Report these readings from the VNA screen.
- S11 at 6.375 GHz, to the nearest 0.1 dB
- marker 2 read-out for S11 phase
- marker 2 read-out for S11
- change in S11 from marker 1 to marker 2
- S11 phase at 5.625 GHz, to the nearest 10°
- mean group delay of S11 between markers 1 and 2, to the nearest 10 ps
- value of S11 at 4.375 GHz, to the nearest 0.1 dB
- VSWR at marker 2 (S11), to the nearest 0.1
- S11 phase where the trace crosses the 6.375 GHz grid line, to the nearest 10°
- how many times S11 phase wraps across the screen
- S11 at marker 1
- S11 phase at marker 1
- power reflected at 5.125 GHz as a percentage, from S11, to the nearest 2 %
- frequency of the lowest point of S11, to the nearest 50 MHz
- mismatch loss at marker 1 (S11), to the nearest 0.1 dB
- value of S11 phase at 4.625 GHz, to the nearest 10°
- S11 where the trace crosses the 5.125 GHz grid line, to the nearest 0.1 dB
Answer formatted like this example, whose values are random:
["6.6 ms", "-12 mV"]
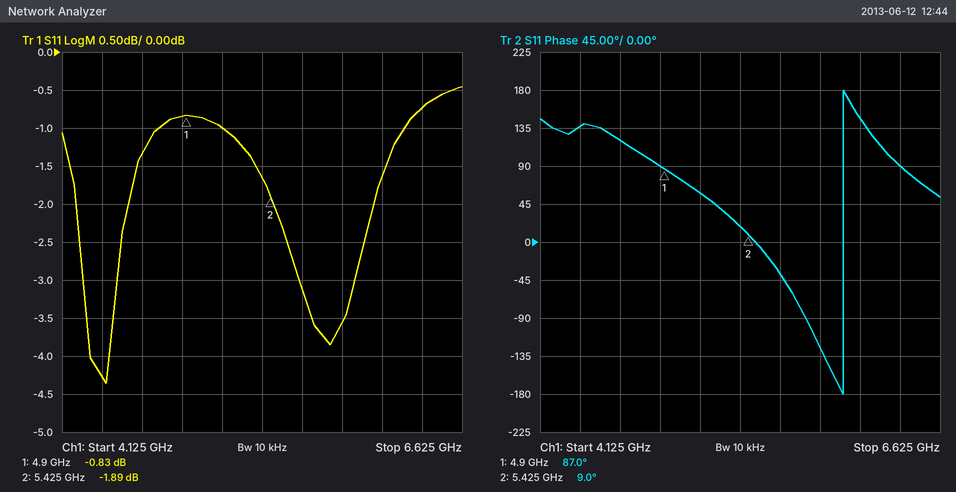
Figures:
["-0.7 dB", "9.0°", "-1.89 dB", "-1.06 dB", "-40°", "410 ps", "-4.3 dB", "9.2", "90°", "1", "-0.83 dB", "87.0°", "80 %", "4.40 GHz", "7.6 dB", "120°", "-1.0 dB"]
